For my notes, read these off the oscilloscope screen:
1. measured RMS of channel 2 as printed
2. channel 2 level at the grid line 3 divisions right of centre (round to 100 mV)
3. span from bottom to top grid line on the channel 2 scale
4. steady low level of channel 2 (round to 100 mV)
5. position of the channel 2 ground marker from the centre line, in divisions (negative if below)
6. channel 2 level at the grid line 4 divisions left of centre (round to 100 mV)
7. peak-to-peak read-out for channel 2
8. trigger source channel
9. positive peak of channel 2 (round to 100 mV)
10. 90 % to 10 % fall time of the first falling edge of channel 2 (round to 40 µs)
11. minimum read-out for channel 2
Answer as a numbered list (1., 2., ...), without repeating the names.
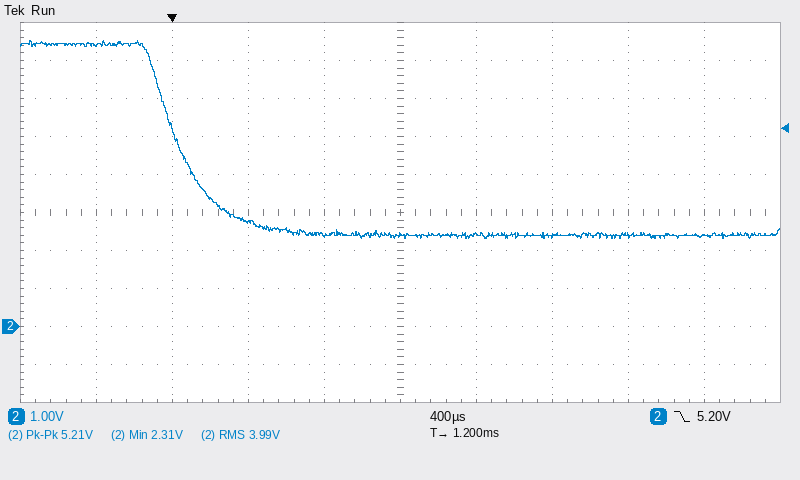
1. 3.99 V
2. 2.4 V
3. 10 V
4. 2.4 V
5. -3.0 div
6. 7.4 V
7. 5.21 V
8. channel 2
9. 7.5 V
10. 440 µs
11. 2.31 V
